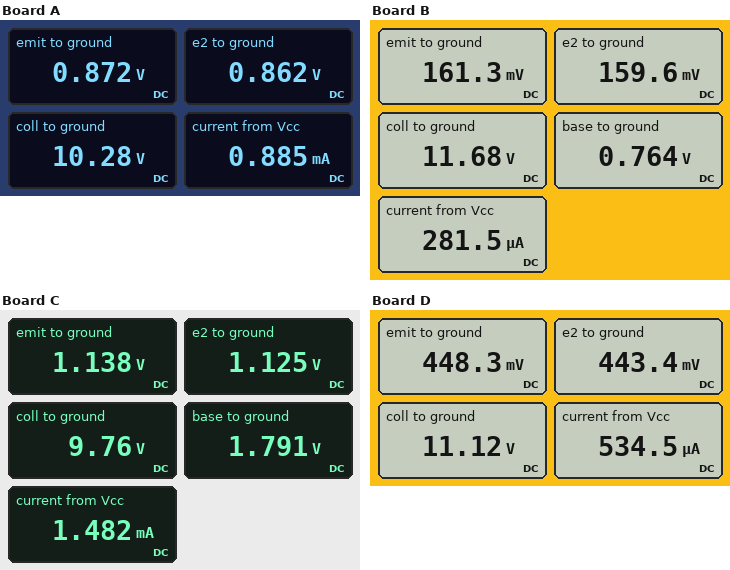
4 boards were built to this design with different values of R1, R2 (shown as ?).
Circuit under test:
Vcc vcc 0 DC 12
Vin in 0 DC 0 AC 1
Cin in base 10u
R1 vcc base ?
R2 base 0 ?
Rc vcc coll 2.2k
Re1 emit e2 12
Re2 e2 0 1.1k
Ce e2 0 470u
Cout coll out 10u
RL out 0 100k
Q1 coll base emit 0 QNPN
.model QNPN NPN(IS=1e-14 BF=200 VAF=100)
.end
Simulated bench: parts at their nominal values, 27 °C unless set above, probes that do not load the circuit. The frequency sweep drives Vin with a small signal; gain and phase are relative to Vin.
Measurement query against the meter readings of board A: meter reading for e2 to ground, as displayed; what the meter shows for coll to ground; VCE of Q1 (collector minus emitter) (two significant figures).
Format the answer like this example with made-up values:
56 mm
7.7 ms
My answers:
0.862 V
10.28 V
9.4 V
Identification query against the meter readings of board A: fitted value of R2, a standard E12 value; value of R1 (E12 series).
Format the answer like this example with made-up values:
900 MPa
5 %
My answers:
15 kΩ
100 kΩ
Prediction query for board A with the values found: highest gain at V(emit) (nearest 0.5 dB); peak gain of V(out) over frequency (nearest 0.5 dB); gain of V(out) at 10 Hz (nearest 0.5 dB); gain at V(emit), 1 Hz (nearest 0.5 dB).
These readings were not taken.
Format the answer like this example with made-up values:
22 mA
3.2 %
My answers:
-3.0 dB
33.5 dB
30.5 dB
-5.5 dB
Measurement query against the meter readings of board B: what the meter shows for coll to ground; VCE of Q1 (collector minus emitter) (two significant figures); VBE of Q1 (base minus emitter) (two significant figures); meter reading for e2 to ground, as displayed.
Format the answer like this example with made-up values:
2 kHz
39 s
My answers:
11.68 V
12 V
600 mV
159.6 mV
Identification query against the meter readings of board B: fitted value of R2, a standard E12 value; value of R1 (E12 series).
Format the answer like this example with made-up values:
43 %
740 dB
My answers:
5.6 kΩ
82 kΩ
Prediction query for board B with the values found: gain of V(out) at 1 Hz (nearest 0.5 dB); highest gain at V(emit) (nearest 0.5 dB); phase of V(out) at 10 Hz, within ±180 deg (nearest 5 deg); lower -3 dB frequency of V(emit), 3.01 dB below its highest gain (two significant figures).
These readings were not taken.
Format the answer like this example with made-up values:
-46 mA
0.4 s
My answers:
3.5 dB
-9.5 dB
-150 deg
1.0 Hz
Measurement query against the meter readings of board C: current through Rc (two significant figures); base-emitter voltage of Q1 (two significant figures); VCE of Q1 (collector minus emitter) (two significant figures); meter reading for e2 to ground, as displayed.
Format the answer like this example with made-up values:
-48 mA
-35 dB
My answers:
1.0 mA
650 mV
8.6 V
1.125 V
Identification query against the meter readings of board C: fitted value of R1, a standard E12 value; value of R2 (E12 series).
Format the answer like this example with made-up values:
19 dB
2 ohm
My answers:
22 kΩ
3.9 kΩ
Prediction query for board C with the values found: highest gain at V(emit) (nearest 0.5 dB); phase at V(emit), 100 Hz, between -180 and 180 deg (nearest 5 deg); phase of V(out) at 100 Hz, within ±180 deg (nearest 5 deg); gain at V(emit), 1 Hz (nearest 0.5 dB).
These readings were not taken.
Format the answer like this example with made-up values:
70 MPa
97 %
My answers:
-4.5 dB
-5 deg
-170 deg
-14.5 dB
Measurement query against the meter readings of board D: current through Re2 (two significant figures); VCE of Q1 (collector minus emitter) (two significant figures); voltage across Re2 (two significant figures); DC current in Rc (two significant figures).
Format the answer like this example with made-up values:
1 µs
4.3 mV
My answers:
400 µA
11 V
440 mV
400 µA
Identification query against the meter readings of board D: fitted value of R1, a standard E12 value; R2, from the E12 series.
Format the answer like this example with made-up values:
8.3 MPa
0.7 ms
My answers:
82 kΩ
8.2 kΩ
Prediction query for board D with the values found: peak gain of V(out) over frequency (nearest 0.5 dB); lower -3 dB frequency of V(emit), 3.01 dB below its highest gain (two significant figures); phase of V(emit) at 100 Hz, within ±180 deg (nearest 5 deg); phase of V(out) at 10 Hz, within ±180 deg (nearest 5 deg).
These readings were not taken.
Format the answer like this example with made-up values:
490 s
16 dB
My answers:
29.0 dB
1.2 Hz
-10 deg
-140 deg
